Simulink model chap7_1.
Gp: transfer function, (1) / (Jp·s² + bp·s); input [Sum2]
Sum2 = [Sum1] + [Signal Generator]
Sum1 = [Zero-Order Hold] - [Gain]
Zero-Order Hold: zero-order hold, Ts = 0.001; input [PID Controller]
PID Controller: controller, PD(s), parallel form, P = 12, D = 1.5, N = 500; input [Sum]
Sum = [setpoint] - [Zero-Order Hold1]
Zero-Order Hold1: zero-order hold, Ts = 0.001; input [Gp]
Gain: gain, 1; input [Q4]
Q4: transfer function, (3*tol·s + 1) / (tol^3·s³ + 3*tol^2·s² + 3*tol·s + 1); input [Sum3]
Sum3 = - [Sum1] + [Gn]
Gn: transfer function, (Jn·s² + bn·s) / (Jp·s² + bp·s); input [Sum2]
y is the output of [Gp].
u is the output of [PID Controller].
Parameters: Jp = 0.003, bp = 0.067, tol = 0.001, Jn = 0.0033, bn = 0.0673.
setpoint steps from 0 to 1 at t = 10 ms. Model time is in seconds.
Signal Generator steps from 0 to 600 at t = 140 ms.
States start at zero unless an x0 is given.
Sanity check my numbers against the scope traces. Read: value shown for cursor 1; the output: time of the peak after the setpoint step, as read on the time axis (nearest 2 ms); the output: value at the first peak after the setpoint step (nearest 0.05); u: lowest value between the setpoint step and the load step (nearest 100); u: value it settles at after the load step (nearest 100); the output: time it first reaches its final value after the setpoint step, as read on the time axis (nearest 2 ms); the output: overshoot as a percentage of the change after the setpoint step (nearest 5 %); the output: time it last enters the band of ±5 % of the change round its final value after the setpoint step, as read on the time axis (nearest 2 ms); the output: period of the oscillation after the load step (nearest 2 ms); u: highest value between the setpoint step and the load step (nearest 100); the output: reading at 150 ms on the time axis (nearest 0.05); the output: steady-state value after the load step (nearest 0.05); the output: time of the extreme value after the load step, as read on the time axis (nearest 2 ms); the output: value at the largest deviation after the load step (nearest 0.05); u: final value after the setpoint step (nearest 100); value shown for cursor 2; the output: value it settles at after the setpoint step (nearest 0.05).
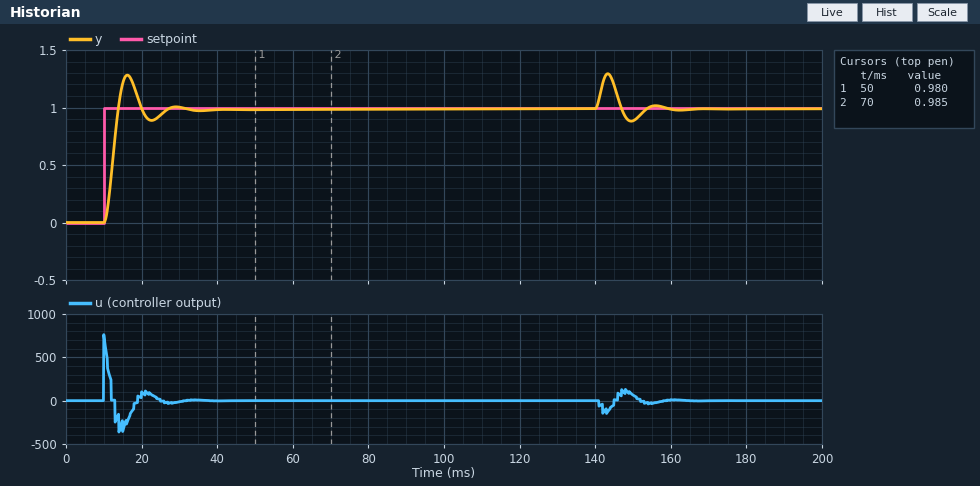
0.980
16 ms
1.30
-400
0
14 ms
30 %
26 ms
12 ms
800
0.90
1.00
144 ms
1.30
0
0.985
1.00
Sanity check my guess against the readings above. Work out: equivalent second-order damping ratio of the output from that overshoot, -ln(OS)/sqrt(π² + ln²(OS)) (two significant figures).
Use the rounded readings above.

0.36
